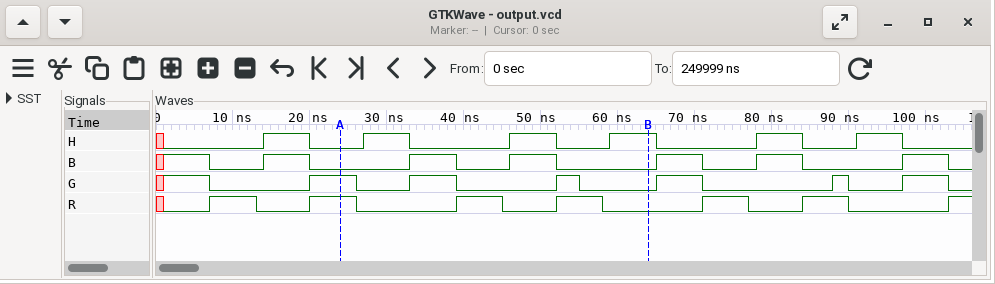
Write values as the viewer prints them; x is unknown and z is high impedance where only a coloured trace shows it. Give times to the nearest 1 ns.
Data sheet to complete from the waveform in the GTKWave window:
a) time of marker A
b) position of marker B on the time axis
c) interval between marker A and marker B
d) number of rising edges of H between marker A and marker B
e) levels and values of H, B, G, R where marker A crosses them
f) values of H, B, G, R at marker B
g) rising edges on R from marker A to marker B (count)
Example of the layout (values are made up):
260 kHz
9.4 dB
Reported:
24 ns
64 ns
40 ns
3
H=0, B=0, G=1, R=1
H=1, B=0, G=0, R=0
2
